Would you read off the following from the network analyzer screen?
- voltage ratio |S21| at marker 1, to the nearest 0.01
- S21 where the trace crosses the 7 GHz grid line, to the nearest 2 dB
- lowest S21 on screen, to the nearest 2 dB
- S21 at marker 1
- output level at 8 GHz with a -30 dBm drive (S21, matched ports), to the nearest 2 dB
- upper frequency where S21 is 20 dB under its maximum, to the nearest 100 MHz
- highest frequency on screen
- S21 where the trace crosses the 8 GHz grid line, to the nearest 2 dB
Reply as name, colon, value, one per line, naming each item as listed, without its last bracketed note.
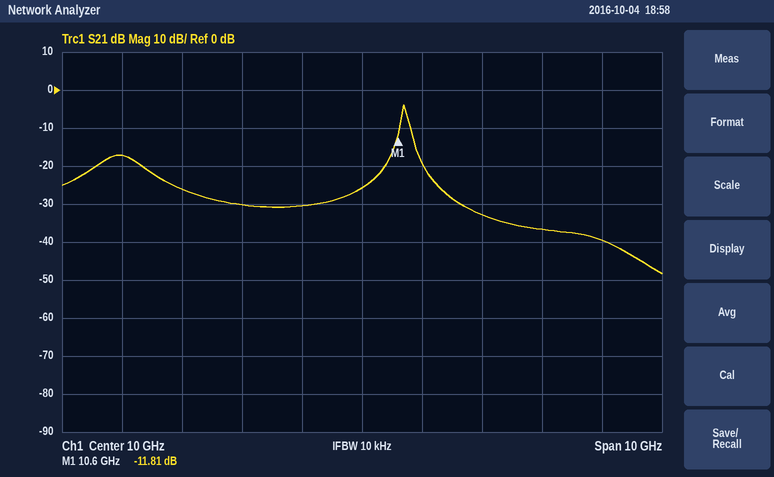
voltage ratio |S21| at marker 1, to the nearest 0.01: 0.26
S21 where the trace crosses the 7 GHz grid line, to the nearest 2 dB: -26 dB
lowest S21 on screen, to the nearest 2 dB: -48 dB
S21 at marker 1: -11.81 dB
output level at 8 GHz with a -30 dBm drive (S21, matched ports), to the nearest 2 dB: -60 dBm
upper frequency where S21 is 20 dB under its maximum, to the nearest 100 MHz: 11.2 GHz
highest frequency on screen: 15 GHz
S21 where the trace crosses the 8 GHz grid line, to the nearest 2 dB: -30 dB
